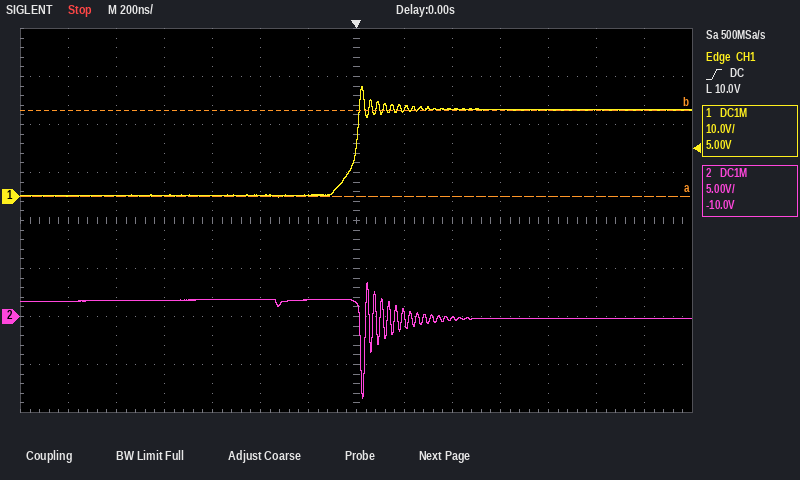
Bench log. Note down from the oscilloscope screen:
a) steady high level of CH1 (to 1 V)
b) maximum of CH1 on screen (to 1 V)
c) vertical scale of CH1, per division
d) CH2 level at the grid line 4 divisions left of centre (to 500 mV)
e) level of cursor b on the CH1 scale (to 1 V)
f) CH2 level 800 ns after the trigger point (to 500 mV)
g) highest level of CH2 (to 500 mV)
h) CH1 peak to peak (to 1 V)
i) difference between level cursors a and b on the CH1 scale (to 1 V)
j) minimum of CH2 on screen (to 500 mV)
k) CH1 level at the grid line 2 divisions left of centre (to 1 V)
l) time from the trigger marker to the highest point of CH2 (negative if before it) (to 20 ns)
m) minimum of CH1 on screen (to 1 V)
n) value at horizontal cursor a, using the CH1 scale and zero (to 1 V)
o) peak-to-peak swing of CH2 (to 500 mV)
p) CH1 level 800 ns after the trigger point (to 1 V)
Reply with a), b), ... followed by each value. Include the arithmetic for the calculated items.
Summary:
a) 18 V
b) 23 V
c) 10 V
d) 1.5 V
e) 18 V
f) 0.0 V
g) 3.5 V
h) 23 V − (0 V) = 23 V
i) 18 V
j) -8.5 V
k) 0 V
l) +40 ns
m) 0 V
n) 0 V
o) 3.5 V − (-8.5 V) = 12.0 V
p) 18 V
